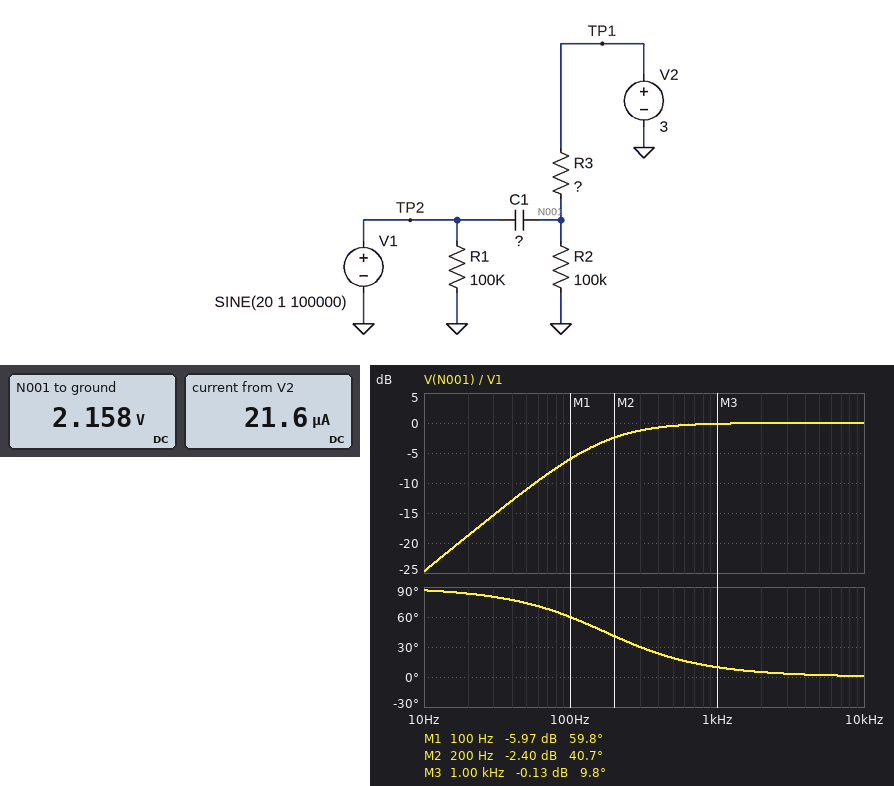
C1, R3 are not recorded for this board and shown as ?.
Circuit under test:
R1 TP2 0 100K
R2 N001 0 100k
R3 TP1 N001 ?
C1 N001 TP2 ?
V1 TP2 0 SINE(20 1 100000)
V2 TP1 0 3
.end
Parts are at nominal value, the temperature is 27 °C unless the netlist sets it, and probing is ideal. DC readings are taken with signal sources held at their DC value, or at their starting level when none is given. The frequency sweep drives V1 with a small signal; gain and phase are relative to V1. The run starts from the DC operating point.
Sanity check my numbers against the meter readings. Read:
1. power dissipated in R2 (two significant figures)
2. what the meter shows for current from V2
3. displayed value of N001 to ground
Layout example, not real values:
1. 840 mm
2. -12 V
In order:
1. 47 µW
2. 21.6 µA
3. 2.158 V
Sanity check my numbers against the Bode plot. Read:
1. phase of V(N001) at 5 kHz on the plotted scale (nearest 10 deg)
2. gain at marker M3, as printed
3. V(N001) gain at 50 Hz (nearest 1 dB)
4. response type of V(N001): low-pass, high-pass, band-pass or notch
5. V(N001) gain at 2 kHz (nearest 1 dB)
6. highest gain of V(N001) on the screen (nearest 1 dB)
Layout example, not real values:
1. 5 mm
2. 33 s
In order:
1. 0 deg
2. -0.13 dB
3. -11 dB
4. high-pass
5. 0 dB
6. 0 dB
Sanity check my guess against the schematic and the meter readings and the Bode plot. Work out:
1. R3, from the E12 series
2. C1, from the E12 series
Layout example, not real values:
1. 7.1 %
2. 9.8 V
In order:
1. 39 kΩ
2. 33 nF
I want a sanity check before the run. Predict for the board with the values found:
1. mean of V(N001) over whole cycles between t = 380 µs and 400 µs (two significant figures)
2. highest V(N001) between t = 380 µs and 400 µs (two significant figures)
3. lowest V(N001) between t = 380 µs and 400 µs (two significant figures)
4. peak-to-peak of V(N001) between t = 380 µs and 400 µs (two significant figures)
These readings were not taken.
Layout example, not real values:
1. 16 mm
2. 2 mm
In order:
1. 2.2 V
2. 3.2 V
3. 1.2 V
4. 2.0 V
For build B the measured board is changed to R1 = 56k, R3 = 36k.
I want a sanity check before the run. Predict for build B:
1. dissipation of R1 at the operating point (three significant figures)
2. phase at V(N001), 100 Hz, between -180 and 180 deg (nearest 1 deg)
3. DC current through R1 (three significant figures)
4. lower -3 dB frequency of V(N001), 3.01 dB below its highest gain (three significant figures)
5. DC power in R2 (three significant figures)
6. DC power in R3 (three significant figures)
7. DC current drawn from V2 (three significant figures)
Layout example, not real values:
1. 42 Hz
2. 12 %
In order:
1. 7.14 mW
2. 61 deg
3. 357 µA
4. 182 Hz
5. 48.7 µW
6. 17.5 µW
7. 22.1 µA
